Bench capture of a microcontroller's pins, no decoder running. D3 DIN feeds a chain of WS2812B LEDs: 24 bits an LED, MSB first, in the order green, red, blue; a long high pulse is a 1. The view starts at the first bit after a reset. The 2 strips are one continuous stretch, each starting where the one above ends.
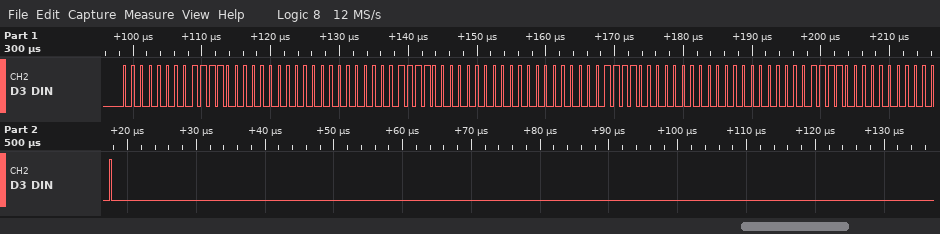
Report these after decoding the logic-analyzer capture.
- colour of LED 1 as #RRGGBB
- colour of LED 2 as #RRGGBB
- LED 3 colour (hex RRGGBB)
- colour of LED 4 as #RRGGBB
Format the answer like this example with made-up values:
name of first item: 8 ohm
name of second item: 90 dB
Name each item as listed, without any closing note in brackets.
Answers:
colour of LED 1 as #RRGGBB: #F00000
colour of LED 2 as #RRGGBB: #F00000
LED 3 colour: #F00000
colour of LED 4 as #RRGGBB: #F00000
